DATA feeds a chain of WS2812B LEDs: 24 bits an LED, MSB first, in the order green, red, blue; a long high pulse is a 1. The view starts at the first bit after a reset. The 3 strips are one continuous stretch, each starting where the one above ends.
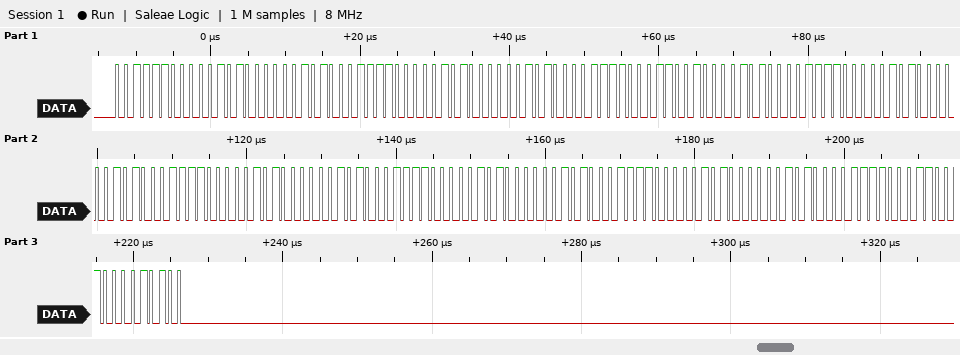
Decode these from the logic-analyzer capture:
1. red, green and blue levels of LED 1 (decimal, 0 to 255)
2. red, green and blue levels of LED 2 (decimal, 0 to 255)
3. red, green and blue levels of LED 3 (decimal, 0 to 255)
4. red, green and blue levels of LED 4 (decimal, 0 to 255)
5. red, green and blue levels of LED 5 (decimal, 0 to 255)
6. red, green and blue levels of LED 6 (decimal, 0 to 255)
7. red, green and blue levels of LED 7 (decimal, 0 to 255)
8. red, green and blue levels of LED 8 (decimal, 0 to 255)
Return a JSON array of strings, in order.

["20, 60, 10", "20, 60, 10", "50, 30, 20", "20, 60, 10", "20, 60, 10", "20, 60, 10", "20, 60, 10", "50, 30, 20"]
